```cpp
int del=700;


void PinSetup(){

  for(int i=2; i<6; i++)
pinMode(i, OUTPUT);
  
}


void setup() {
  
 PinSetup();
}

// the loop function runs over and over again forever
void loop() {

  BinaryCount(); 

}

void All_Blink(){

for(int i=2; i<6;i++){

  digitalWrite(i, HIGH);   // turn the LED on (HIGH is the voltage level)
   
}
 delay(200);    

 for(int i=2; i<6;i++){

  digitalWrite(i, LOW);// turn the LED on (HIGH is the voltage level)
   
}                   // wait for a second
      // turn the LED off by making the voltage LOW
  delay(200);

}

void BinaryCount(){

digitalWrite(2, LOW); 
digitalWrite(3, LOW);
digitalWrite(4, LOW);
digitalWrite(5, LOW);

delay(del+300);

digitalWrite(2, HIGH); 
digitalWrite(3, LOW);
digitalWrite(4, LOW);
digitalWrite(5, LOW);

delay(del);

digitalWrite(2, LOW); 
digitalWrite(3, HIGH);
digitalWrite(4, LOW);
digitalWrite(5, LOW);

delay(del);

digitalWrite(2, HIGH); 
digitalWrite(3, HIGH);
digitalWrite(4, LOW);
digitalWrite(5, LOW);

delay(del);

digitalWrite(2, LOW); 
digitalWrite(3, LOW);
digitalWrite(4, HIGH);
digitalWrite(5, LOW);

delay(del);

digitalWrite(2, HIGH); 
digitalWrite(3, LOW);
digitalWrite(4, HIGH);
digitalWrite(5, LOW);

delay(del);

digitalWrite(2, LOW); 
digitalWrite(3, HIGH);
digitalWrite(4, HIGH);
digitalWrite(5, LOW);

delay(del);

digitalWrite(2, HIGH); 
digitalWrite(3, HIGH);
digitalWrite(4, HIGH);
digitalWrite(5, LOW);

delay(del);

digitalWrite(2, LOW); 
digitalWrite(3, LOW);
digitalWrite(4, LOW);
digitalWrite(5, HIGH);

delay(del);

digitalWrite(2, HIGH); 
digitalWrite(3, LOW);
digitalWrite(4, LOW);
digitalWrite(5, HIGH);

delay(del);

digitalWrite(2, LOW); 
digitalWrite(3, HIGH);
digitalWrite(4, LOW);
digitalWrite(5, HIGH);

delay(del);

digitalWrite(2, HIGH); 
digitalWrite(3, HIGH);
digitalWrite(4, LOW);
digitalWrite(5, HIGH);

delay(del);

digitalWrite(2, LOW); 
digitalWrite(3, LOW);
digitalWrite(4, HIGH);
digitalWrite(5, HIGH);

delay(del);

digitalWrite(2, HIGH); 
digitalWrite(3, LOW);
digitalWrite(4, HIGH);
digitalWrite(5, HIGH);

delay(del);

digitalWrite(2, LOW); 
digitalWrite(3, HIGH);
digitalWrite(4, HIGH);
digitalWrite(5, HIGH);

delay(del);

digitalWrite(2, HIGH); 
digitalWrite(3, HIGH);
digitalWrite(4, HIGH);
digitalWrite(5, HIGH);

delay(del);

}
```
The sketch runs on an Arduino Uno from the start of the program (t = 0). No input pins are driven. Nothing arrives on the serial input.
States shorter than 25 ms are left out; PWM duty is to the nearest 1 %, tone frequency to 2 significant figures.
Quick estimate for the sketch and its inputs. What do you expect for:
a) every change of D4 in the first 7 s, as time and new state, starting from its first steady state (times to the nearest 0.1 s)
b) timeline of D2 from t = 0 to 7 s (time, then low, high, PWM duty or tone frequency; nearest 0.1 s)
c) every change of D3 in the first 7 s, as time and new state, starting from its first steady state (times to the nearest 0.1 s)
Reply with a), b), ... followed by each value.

a) 0 s low; 3.1 s high; 5.9 s low
b) 0 s low; 1 s high; 1.7 s low; 2.4 s high; 3.1 s low; 3.8 s high; 4.5 s low; 5.2 s high; 5.9 s low; 6.6 s high
c) 0 s low; 1.7 s high; 3.1 s low; 4.5 s high; 5.9 s low
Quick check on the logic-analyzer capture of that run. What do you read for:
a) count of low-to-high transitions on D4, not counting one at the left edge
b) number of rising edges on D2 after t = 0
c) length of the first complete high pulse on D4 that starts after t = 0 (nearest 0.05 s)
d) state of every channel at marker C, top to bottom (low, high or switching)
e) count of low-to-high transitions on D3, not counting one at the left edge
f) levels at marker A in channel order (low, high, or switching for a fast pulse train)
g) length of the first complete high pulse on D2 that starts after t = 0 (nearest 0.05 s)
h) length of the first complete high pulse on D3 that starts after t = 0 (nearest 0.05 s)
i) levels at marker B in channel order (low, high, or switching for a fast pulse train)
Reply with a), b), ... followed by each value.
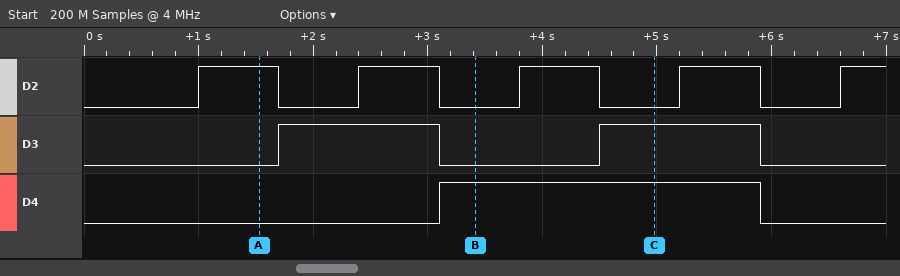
a) 1
b) 5
c) 2.80 s
d) D2 low, D3 high, D4 high
e) 2
f) D2 high, D3 low, D4 low
g) 0.70 s
h) 1.40 s
i) D2 low, D3 low, D4 high
